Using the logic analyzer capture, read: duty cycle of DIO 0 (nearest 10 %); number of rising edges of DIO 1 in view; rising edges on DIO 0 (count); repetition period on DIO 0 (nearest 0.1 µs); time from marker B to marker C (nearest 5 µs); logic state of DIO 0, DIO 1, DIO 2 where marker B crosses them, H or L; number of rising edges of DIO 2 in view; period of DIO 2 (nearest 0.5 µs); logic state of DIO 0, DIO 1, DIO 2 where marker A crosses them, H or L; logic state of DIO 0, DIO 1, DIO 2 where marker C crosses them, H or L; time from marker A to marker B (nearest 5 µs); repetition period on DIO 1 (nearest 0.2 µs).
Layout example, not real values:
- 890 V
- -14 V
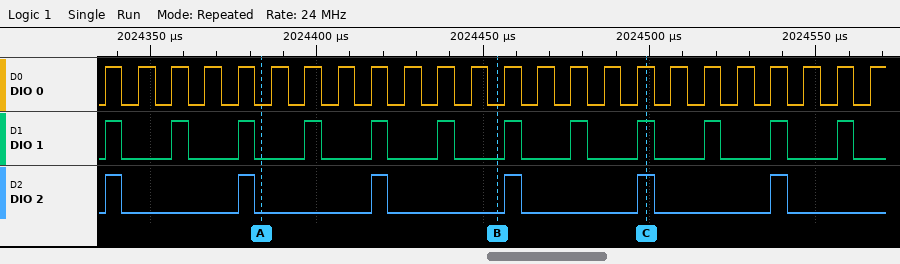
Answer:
- 50 %
- 12
- 24
- 10 µs
- 45 µs
- DIO 0=L, DIO 1=L, DIO 2=L
- 6
- 40 µs
- DIO 0=L, DIO 1=L, DIO 2=L
- DIO 0=H, DIO 1=H, DIO 2=H
- 70 µs
- 20 µs
